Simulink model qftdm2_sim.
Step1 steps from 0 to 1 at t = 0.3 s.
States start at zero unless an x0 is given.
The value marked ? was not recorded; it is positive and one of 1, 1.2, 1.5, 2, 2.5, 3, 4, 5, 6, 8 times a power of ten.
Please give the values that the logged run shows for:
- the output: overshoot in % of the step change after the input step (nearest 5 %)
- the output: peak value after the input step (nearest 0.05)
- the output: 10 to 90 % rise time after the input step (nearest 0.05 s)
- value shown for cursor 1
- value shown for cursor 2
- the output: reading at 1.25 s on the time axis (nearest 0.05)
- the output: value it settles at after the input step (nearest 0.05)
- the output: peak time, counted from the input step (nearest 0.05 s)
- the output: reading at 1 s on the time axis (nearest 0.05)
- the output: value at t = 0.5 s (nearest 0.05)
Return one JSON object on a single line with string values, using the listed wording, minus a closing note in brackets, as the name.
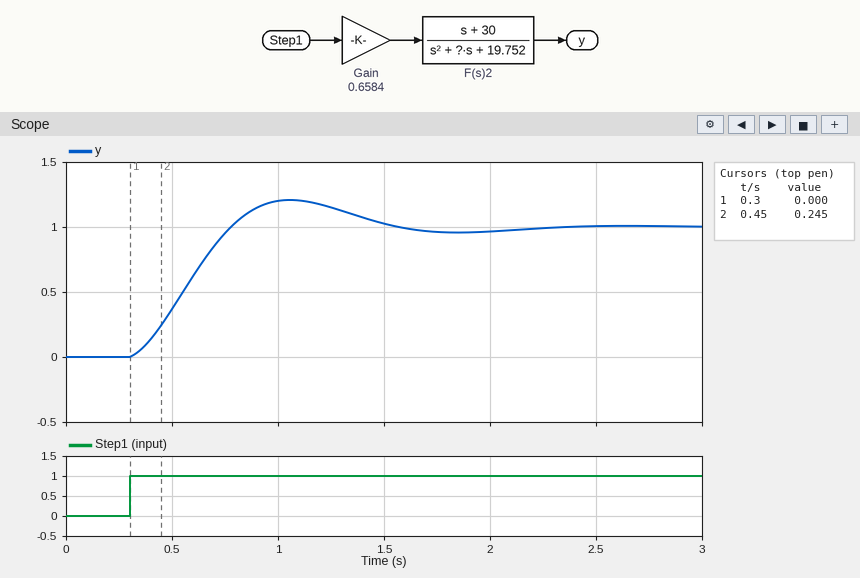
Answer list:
{"the output: overshoot in % of the step change after the input step": "20 %", "the output: peak value after the input step": "1.20", "the output: 10 to 90 % rise time after the input step": "0.35 s", "value shown for cursor 1": "0.000", "value shown for cursor 2": "0.245", "the output: reading at 1.25 s on the time axis": "1.15", "the output: value it settles at after the input step": "1.00", "the output: peak time, counted from the input step": "0.75 s", "the output: reading at 1 s on the time axis": "1.20", "the output: value at t = 0.5 s": "0.35"}
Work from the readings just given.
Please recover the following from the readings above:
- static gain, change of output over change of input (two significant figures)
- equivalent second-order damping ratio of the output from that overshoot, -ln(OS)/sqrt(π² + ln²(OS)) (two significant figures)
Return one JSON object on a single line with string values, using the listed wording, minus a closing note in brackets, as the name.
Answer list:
{"static gain, change of output over change of input": "1.0", "equivalent second-order damping ratio of the output from that overshoot, -ln(OS)/sqrt(π² + ln²(OS))": "0.46"}
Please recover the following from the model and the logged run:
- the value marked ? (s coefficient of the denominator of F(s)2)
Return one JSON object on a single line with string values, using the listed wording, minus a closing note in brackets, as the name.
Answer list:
{"the value marked ? (s coefficient of the denominator of F(s)2)": "4"}
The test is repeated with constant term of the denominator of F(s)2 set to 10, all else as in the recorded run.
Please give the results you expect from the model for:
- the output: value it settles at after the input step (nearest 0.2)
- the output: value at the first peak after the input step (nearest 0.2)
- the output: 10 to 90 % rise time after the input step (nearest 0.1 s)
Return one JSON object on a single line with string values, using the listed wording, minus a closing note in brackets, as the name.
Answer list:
{"the output: value it settles at after the input step": "2.0", "the output: value at the first peak after the input step": "2.2", "the output: 10 to 90 % rise time after the input step": "0.6 s"}
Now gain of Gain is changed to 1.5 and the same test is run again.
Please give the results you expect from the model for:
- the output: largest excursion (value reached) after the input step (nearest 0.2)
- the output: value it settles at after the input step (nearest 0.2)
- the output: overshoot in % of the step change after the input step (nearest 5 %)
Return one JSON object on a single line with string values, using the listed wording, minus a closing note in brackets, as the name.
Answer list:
{"the output: largest excursion (value reached) after the input step": "2.8", "the output: value it settles at after the input step": "2.2", "the output: overshoot in % of the step change after the input step": "20 %"}
